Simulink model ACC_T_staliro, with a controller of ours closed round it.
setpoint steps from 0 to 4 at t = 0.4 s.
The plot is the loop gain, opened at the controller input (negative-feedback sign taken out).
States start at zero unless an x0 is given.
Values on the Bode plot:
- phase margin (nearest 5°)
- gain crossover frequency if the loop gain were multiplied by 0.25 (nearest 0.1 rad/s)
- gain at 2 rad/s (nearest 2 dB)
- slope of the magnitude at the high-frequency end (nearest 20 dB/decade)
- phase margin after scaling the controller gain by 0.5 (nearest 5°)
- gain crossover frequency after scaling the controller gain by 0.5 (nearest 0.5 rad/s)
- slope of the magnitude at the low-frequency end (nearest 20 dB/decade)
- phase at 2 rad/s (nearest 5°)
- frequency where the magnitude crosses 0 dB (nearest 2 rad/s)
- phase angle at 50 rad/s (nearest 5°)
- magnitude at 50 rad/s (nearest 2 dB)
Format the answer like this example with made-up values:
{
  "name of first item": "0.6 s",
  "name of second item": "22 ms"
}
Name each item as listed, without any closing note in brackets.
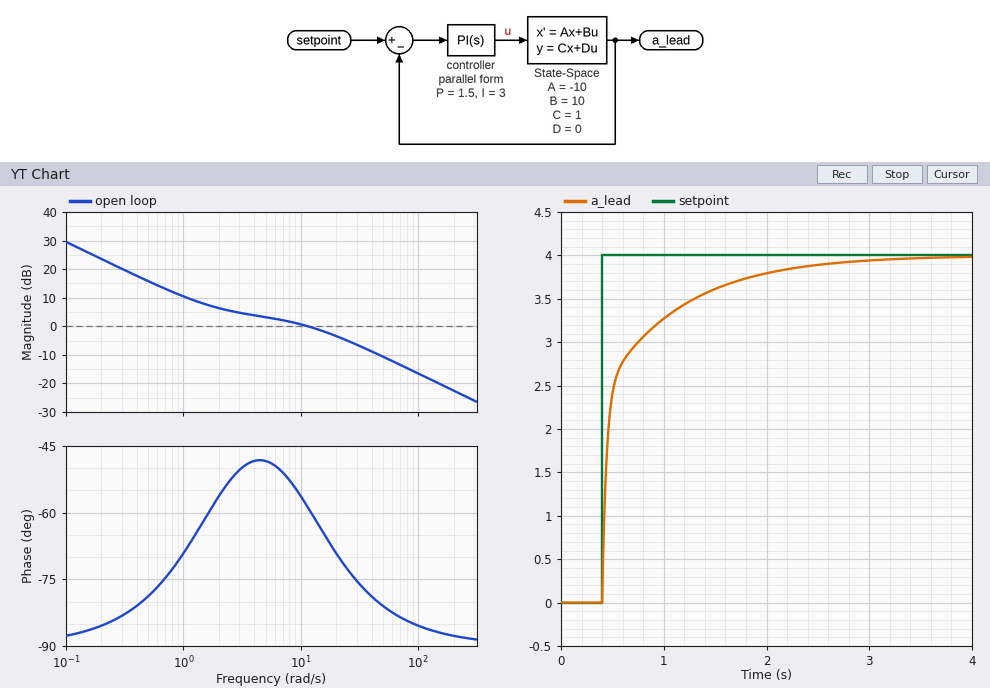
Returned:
{
  "phase margin": "120°",
  "gain crossover frequency if the loop gain were multiplied by 0.25": "0.8 rad/s",
  "gain at 2 rad/s": "6 dB",
  "slope of the magnitude at the high-frequency end": "-20 dB/decade",
  "phase margin after scaling the controller gain by 0.5": "125°",
  "gain crossover frequency after scaling the controller gain by 0.5": "2.0 rad/s",
  "slope of the magnitude at the low-frequency end": "-20 dB/decade",
  "phase at 2 rad/s": "-55°",
  "frequency where the magnitude crosses 0 dB": "12 rad/s",
  "phase angle at 50 rad/s": "-80°",
  "magnitude at 50 rad/s": "-10 dB"
}
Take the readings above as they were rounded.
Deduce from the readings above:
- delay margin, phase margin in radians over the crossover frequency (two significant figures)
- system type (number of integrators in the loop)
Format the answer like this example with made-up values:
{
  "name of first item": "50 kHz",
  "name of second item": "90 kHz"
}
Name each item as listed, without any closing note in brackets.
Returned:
{
  "delay margin, phase margin in radians over the crossover frequency": "0.17 s",
  "system type": "1"
}
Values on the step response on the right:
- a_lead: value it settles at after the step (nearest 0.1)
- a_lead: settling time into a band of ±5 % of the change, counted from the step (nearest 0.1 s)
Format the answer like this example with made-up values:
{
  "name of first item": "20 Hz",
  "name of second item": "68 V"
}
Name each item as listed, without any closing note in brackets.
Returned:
{
  "a_lead: value it settles at after the step": "4.0",
  "a_lead: settling time into a band of ±5 % of the change, counted from the step": "1.6 s"
}
